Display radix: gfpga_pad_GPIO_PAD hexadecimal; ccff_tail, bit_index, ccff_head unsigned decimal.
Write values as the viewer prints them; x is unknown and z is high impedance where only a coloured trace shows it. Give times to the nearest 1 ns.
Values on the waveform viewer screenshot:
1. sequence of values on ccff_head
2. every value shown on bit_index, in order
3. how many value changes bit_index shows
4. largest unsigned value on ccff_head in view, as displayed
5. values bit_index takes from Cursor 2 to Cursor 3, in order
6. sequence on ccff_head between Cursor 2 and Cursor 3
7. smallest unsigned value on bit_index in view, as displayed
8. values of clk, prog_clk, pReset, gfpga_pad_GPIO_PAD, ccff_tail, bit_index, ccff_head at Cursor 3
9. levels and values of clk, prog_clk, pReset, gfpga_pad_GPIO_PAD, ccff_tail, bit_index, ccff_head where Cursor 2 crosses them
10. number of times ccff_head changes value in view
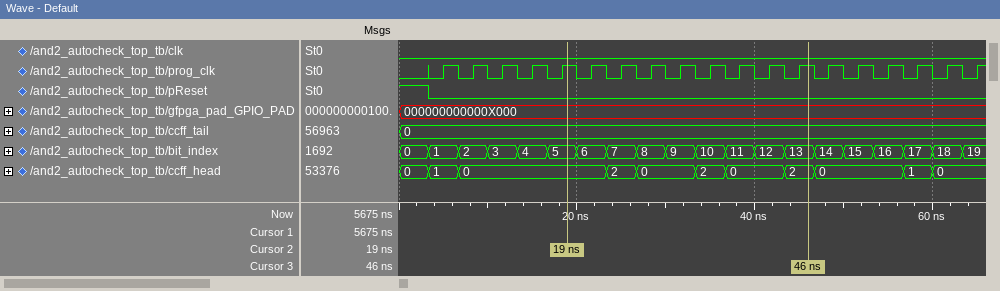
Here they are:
0, 1, 0, 2, 0, 2, 0, 2, 0, 1, 0
0, 1, 2, 3, 4, 5, 6, 7, 8, 9, 10, 11, 12, 13, 14, 15, 16, 17, 18, 19
19
2
5, 6, 7, 8, 9, 10, 11, 12, 13
0, 2, 0, 2, 0, 2
0
clk=0, prog_clk=1, pReset=0, gfpga_pad_GPIO_PAD=000000000000X000, ccff_tail=0, bit_index=13, ccff_head=2
clk=0, prog_clk=1, pReset=0, gfpga_pad_GPIO_PAD=000000000000X000, ccff_tail=0, bit_index=5, ccff_head=0
10
